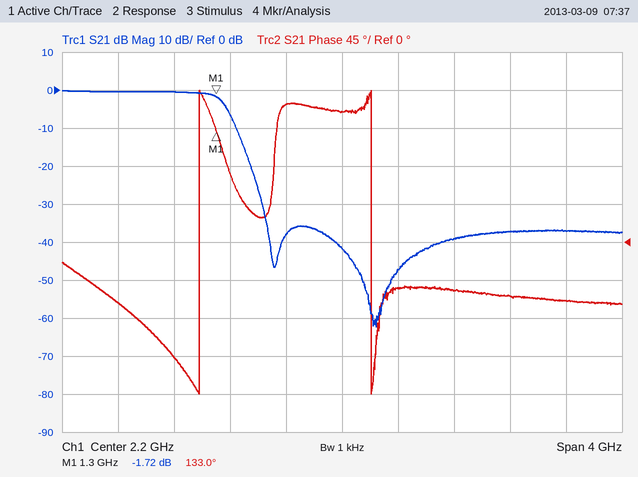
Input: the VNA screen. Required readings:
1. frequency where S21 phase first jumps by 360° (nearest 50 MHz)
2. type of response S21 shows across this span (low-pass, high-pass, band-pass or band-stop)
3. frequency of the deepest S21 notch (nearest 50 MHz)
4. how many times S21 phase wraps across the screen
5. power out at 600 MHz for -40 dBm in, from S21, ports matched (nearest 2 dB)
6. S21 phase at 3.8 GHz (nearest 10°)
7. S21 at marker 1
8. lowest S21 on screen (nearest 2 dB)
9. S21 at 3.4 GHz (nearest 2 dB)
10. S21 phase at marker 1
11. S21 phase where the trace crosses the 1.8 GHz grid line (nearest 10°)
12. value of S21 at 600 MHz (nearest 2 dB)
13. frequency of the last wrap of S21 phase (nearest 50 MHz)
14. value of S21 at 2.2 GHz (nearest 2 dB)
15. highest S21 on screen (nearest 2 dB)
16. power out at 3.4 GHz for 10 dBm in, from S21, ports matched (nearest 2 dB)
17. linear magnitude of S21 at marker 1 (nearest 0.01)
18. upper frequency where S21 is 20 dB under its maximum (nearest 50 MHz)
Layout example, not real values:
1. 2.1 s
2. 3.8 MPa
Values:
1. 1.20 GHz
2. low-pass
3. 2.45 GHz
4. 2
5. -40 dBm
6. -70°
7. -1.72 dB
8. -62 dB
9. -38 dB
10. 133.0°
11. 160°
12. 0 dB
13. 2.40 GHz
14. -42 dB
15. 0 dB
16. -28 dBm
17. 0.82
18. 1.55 GHz
